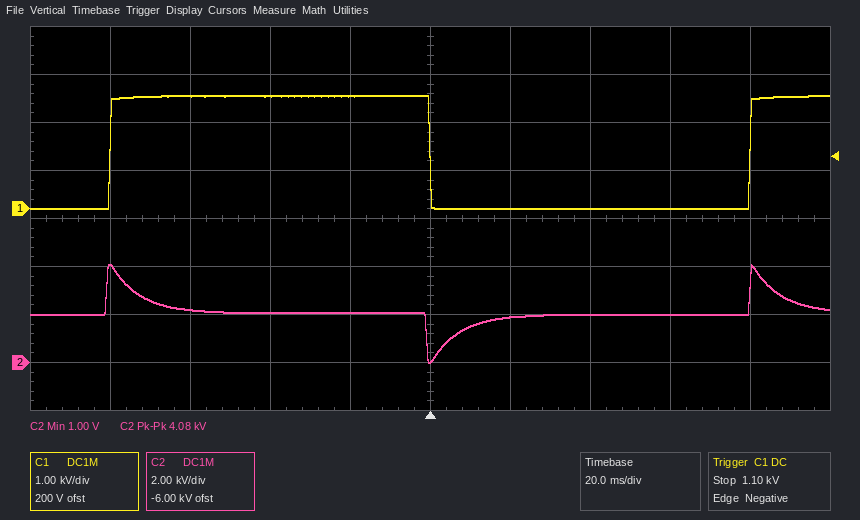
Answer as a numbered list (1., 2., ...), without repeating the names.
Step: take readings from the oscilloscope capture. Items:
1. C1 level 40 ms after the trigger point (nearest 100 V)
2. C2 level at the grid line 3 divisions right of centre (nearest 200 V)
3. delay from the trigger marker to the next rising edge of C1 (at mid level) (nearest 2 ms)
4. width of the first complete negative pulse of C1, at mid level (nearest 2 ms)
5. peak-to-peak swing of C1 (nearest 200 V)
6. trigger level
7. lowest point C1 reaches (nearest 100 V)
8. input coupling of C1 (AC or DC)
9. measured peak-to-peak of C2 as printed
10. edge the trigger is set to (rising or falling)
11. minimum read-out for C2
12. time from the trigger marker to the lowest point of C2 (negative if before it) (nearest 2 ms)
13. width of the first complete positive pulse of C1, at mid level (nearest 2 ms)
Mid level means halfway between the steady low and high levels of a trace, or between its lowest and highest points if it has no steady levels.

1. 0.0 kV
2. 2.0 kV
3. 80 ms
4. 80 ms
5. 2.4 kV
6. 1.10 kV
7. 0.0 kV
8. DC
9. 4.08 kV
10. falling
11. 1.00 V
12. 0 ms
13. 80 ms
